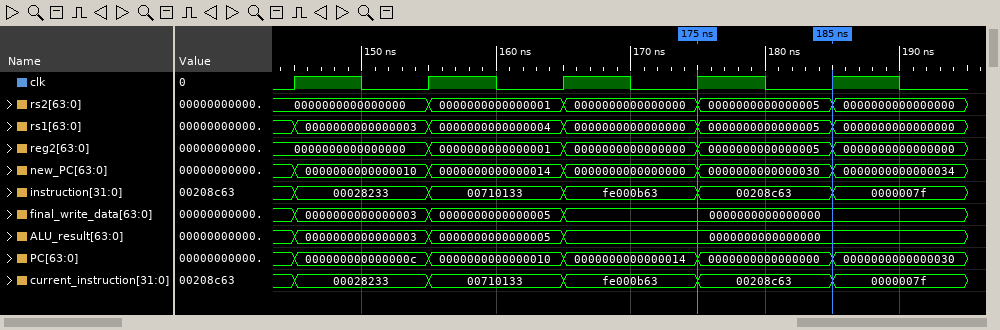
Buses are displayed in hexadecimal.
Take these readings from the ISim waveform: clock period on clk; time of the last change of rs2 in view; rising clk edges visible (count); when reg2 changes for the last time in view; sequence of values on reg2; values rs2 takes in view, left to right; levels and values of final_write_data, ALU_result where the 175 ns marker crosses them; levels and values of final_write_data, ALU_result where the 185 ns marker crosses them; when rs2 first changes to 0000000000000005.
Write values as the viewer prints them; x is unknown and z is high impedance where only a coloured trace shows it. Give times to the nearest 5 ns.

10 ns
185 ns
5
185 ns
0000000000000000, 0000000000000001, 0000000000000000, 0000000000000005, 0000000000000000
0000000000000000, 0000000000000001, 0000000000000000, 0000000000000005, 0000000000000000
final_write_data=0000000000000000, ALU_result=0000000000000000
final_write_data=0000000000000000, ALU_result=0000000000000000
175 ns
